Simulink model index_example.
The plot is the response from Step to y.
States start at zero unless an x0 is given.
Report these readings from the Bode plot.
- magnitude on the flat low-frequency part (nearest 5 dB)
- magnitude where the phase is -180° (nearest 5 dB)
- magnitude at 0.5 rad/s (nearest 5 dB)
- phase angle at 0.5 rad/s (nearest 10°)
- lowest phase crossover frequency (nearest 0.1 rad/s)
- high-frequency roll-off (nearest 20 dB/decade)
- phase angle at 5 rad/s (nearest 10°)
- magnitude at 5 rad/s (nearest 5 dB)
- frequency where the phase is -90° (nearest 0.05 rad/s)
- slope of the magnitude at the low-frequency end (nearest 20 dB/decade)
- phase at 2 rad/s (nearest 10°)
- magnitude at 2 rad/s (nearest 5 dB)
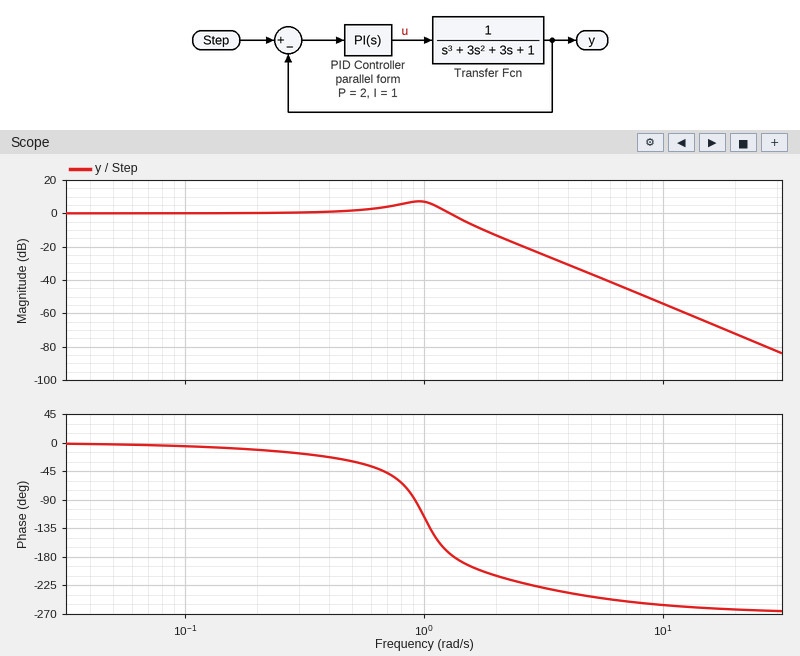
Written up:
0 dB
0 dB
0 dB
-30°
1.3 rad/s
-60 dB/decade
-240°
-35 dB
0.90 rad/s
0 dB/decade
-210°
-15 dB
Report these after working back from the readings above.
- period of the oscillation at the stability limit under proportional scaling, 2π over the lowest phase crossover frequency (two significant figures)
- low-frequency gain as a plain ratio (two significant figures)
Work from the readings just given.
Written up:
4.8 s
1.0
